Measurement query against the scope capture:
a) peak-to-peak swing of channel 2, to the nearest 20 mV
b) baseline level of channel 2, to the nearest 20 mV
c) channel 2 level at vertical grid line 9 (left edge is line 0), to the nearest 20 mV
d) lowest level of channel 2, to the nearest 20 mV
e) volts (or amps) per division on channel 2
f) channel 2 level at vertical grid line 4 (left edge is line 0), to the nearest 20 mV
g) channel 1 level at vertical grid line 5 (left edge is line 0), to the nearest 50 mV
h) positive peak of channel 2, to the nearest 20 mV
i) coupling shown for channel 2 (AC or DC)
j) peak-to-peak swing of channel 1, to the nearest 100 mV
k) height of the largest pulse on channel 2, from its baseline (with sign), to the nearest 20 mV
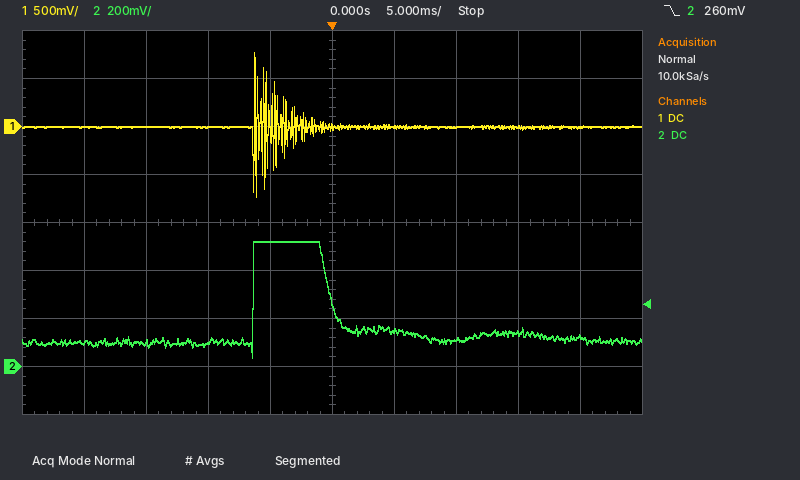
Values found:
480 mV
100 mV
120 mV
40 mV
200 mV
520 mV
0 mV
520 mV
DC
1.50 V
+420 mV
